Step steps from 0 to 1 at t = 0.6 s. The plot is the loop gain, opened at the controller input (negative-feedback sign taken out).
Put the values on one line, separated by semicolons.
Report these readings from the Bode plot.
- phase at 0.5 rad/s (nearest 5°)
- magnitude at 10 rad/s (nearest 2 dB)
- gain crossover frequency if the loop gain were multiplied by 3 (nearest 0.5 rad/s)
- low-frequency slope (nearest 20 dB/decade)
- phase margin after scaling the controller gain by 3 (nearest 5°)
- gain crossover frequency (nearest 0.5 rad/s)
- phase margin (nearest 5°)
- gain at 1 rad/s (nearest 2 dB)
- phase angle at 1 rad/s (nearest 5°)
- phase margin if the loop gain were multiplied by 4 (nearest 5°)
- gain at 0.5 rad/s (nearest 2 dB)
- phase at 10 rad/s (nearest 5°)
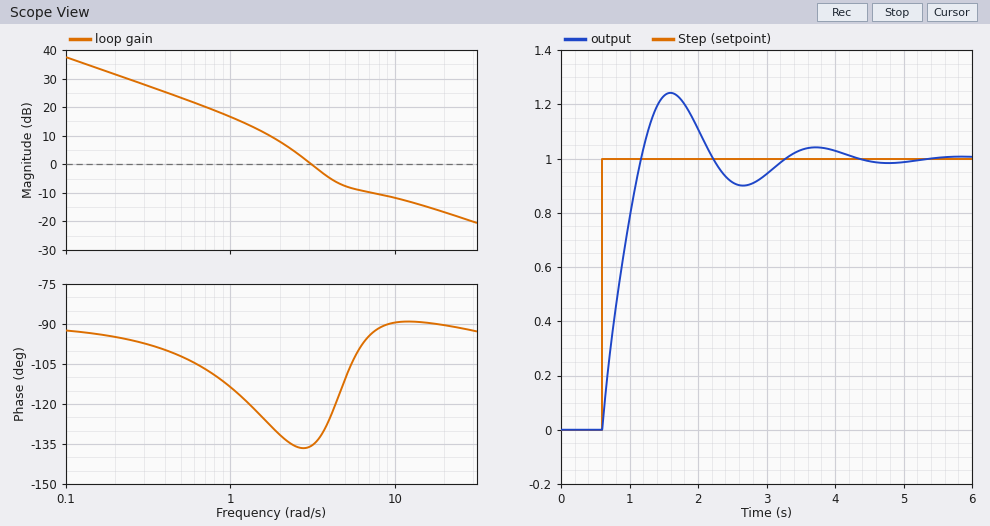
-100°; -12 dB; 6.5 rad/s; -20 dB/decade; 85°; 3.0 rad/s; 45°; 16 dB; -115°; 90°; 24 dB; -90°
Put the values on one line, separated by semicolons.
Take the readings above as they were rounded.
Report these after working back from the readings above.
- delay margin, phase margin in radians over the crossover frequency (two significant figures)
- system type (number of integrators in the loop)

0.26 s; 1
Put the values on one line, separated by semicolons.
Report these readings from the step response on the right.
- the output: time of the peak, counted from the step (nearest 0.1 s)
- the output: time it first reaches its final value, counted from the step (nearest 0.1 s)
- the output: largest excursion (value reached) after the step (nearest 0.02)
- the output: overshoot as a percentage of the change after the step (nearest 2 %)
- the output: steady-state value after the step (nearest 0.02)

1.0 s; 0.6 s; 1.24; 24 %; 1.00
